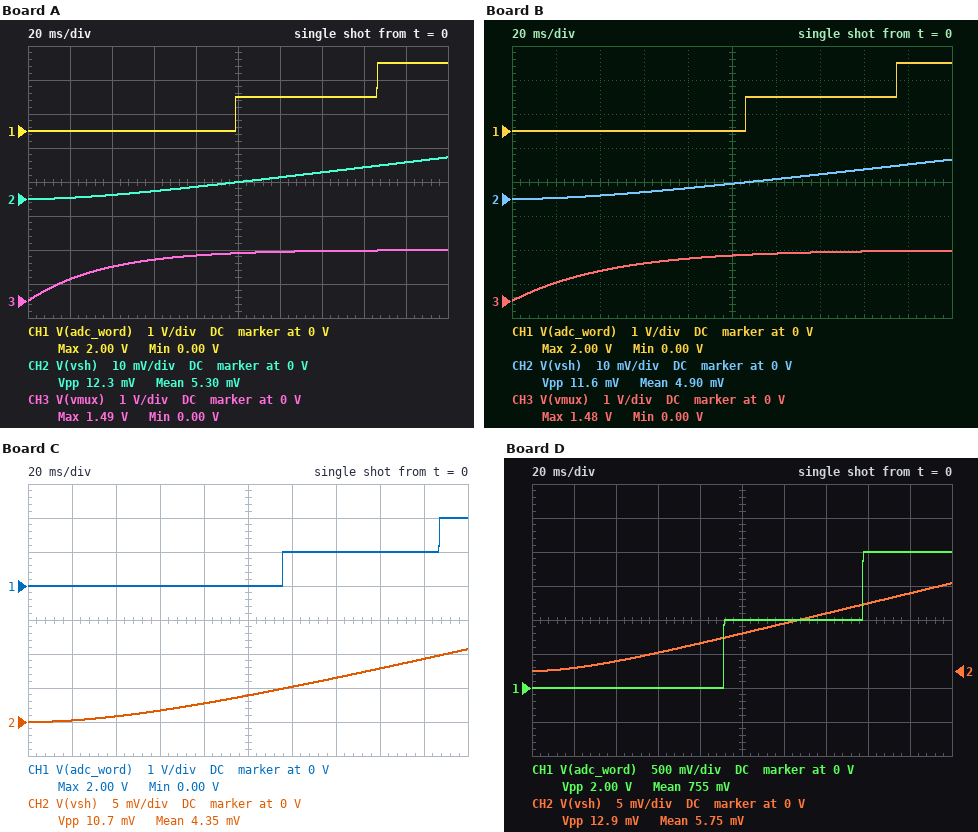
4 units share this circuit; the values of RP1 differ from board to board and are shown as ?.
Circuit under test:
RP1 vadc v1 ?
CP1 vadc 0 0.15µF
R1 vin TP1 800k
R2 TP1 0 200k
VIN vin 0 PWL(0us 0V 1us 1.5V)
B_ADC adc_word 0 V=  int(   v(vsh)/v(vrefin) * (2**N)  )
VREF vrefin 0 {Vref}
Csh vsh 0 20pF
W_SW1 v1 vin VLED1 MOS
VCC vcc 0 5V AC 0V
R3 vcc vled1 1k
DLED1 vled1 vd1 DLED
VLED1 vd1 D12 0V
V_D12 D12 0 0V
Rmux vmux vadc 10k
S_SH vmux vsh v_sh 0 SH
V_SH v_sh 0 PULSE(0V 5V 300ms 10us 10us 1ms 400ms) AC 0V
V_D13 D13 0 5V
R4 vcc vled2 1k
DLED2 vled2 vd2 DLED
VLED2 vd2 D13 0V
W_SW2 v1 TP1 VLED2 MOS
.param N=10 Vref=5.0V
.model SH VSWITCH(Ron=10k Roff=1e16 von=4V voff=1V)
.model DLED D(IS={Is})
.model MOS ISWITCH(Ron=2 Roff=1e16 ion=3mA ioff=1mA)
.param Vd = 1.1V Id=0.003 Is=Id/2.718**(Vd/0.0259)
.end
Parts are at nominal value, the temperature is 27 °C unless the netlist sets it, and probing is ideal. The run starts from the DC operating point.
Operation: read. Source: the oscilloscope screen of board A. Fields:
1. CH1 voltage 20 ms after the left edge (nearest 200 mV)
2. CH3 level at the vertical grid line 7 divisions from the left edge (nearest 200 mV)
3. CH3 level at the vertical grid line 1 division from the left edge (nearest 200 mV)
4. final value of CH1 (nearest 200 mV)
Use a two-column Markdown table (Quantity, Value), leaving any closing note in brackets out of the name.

| Quantity | Value |
|---|---|
| CH1 voltage 20 ms after the left edge | 0 V |
| CH3 level at the vertical grid line 7 divisions from the left edge | 1.4 V |
| CH3 level at the vertical grid line 1 division from the left edge | 600 mV |
| final value of CH1 | 2.0 V |
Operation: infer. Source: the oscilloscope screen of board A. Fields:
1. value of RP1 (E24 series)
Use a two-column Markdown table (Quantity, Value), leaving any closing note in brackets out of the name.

| Quantity | Value |
|---|---|
| value of RP1 | 240 kΩ |
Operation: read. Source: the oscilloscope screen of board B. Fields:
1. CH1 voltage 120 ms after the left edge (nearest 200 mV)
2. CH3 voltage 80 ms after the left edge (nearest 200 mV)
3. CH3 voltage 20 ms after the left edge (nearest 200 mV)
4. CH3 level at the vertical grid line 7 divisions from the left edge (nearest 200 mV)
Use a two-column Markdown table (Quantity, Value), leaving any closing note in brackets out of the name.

| Quantity | Value |
|---|---|
| CH1 voltage 120 ms after the left edge | 1.0 V |
| CH3 voltage 80 ms after the left edge | 1.2 V |
| CH3 voltage 20 ms after the left edge | 600 mV |
| CH3 level at the vertical grid line 7 divisions from the left edge | 1.4 V |
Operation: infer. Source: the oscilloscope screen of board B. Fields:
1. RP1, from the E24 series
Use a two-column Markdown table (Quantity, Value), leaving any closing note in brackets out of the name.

| Quantity | Value |
|---|---|
| RP1, from the E24 series | 300 kΩ |
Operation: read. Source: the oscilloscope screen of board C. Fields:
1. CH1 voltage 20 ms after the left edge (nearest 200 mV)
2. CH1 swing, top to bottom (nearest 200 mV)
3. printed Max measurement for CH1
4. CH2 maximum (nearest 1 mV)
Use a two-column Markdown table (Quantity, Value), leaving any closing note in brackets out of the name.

| Quantity | Value |
|---|---|
| CH1 voltage 20 ms after the left edge | 0 V |
| CH1 swing, top to bottom | 2.0 V |
| printed Max measurement for CH1 | 2.00 V |
| CH2 maximum | 11 mV |
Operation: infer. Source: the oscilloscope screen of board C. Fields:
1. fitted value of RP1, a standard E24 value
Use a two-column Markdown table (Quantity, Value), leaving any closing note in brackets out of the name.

| Quantity | Value |
|---|---|
| fitted value of RP1, a standard E24 value | 390 kΩ |
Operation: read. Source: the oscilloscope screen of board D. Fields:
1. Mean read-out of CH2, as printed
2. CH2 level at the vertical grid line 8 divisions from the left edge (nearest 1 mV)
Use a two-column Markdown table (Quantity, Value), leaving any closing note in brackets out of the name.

| Quantity | Value |
|---|---|
| Mean read-out of CH2, as printed | 5.75 mV |
| CH2 level at the vertical grid line 8 divisions from the left edge | 10 mV |
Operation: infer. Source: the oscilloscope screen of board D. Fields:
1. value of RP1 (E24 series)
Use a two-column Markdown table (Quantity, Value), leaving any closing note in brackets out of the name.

| Quantity | Value |
|---|---|
| value of RP1 | 180 kΩ |
